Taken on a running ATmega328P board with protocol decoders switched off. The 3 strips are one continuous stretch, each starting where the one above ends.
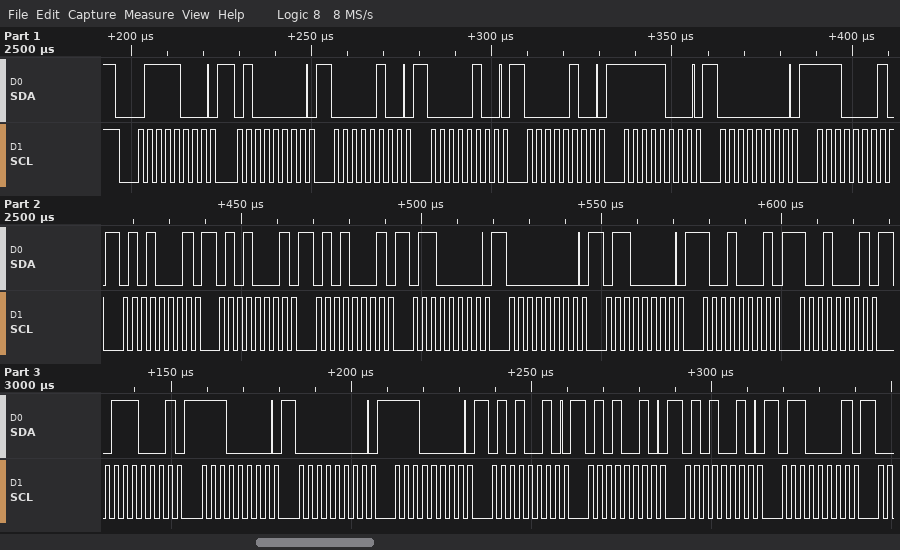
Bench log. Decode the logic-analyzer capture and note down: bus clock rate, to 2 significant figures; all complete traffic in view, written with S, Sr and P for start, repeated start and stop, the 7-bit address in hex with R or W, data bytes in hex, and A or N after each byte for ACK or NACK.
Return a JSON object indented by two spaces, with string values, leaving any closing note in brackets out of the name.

{
  "bus clock rate, to 2 significant figures": "400 kHz",
  "all complete traffic in view, written with S, Sr and P for start, repeated start and stop, the 7-bit address in hex with R or W, data bytes in hex, and A or N after each byte for ACK or NACK": "S 3CW A 40 A 04 A 04 A 04 A F8 A 00 A E1 A 51 A 51 A 51 A 60 A 00 A 60 A 91 A 91 A 71 A E0 A 00 A E0 A 52 A 52 A 52 A 61 A"
}
